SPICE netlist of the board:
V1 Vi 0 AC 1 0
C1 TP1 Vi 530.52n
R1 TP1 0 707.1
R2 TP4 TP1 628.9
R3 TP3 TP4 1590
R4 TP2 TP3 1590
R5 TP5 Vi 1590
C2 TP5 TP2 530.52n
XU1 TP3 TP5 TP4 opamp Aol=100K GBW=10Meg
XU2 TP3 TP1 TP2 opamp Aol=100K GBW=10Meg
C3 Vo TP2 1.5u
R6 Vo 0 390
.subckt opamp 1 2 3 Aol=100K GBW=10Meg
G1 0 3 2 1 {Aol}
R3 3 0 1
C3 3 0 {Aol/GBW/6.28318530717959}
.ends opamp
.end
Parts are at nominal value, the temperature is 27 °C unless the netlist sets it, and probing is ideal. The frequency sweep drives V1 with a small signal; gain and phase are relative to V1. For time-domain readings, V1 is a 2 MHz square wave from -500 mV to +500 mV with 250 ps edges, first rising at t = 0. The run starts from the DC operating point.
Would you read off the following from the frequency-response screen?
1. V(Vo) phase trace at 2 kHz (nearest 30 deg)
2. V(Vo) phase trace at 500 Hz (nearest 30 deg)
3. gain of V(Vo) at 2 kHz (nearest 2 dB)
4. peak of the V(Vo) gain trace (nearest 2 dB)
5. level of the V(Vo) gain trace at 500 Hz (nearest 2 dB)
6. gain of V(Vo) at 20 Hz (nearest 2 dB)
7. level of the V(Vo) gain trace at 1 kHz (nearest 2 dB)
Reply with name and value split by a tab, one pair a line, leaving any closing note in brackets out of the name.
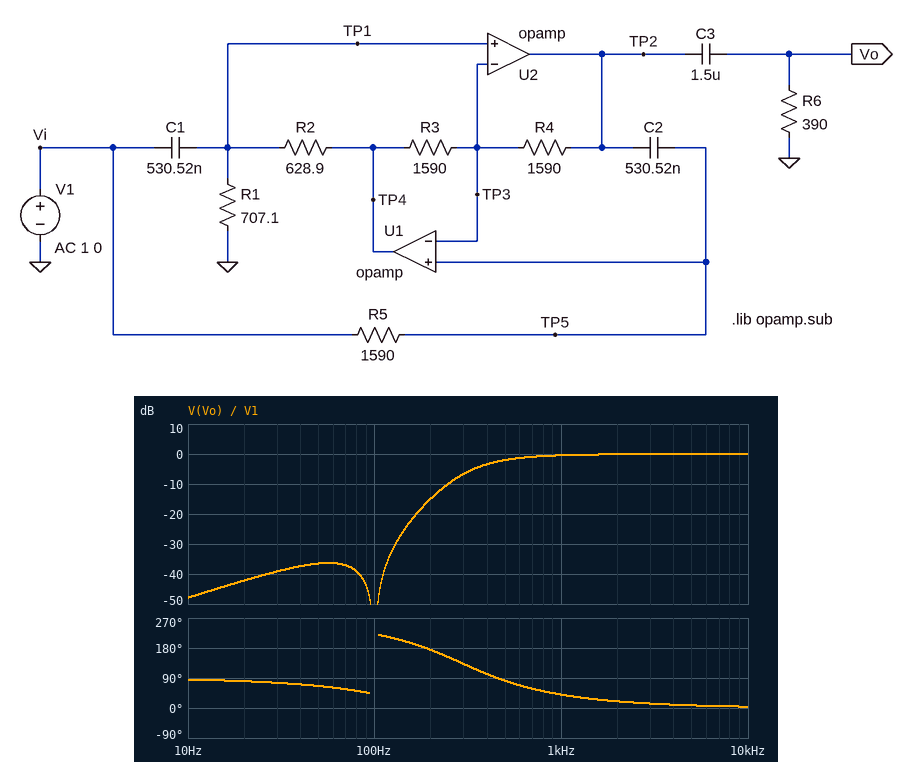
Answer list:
V(Vo) phase trace at 2 kHz	30 deg
V(Vo) phase trace at 500 Hz	90 deg
gain of V(Vo) at 2 kHz	0 dB
peak of the V(Vo) gain trace	0 dB
level of the V(Vo) gain trace at 500 Hz	-2 dB
gain of V(Vo) at 20 Hz	-42 dB
level of the V(Vo) gain trace at 1 kHz	0 dB
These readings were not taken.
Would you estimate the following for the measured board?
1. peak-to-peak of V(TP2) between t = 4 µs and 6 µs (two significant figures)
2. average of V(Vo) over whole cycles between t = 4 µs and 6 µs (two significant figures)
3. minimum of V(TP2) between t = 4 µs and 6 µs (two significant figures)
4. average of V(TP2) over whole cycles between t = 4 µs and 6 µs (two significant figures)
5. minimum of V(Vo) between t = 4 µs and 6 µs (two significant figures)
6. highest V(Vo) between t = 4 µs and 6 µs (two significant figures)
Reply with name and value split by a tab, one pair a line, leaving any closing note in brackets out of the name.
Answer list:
peak-to-peak of V(TP2) between t = 4 µs and 6 µs	1.4 V
average of V(Vo) over whole cycles between t = 4 µs and 6 µs	490 mV
minimum of V(TP2) between t = 4 µs and 6 µs	-270 mV
average of V(TP2) over whole cycles between t = 4 µs and 6 µs	440 mV
minimum of V(Vo) between t = 4 µs and 6 µs	-220 mV
highest V(Vo) between t = 4 µs and 6 µs	1.2 V
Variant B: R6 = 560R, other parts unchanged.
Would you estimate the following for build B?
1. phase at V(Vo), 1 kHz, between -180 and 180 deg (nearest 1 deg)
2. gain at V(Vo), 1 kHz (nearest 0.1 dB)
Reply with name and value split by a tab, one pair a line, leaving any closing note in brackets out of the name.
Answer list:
phase at V(Vo), 1 kHz, between -180 and 180 deg	36 deg
gain at V(Vo), 1 kHz	-0.3 dB
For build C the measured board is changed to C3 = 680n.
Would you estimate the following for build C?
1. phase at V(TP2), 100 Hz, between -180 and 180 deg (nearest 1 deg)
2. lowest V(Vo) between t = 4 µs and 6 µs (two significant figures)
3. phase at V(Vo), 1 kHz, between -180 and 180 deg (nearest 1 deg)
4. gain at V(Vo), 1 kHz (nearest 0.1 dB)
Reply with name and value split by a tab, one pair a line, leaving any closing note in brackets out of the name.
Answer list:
phase at V(TP2), 100 Hz, between -180 and 180 deg	152 deg
lowest V(Vo) between t = 4 µs and 6 µs	-230 mV
phase at V(Vo), 1 kHz, between -180 and 180 deg	56 deg
gain at V(Vo), 1 kHz	-1.5 dB
